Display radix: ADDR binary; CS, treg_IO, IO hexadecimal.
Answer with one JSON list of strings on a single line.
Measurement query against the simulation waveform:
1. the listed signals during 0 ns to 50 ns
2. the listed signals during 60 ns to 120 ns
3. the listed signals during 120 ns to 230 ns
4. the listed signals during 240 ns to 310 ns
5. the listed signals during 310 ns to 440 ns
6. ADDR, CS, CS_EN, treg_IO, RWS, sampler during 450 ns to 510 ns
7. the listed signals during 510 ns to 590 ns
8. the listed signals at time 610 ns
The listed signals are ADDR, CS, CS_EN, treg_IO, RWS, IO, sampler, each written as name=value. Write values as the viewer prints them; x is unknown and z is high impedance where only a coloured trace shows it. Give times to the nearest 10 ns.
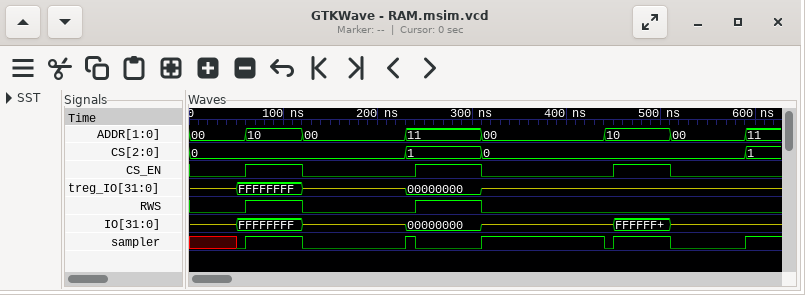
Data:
["ADDR=00, CS=0, CS_EN=0, treg_IO=z, RWS=0, IO=z, sampler=x", "ADDR=10, CS=0, CS_EN=1, treg_IO=FFFFFFFF, RWS=1, IO=FFFFFFFF, sampler=1", "ADDR=00, CS=0, CS_EN=0, treg_IO=z, RWS=0, IO=z, sampler=0", "ADDR=11, CS=1, CS_EN=1, treg_IO=00000000, RWS=1, IO=00000000, sampler=0", "ADDR=00, CS=0, CS_EN=0, treg_IO=z, RWS=0, IO=z, sampler=1", "ADDR=10, CS=0, CS_EN=1, treg_IO=z, RWS=0, sampler=1", "ADDR=00, CS=0, CS_EN=0, treg_IO=z, RWS=0, IO=z, sampler=0", "ADDR=11, CS=1, CS_EN=0, treg_IO=z, RWS=0, IO=z, sampler=1"]
